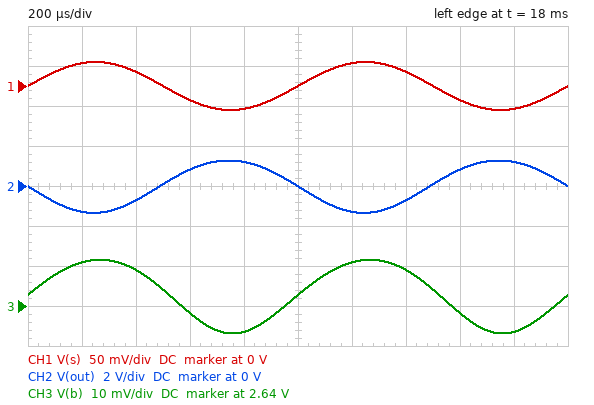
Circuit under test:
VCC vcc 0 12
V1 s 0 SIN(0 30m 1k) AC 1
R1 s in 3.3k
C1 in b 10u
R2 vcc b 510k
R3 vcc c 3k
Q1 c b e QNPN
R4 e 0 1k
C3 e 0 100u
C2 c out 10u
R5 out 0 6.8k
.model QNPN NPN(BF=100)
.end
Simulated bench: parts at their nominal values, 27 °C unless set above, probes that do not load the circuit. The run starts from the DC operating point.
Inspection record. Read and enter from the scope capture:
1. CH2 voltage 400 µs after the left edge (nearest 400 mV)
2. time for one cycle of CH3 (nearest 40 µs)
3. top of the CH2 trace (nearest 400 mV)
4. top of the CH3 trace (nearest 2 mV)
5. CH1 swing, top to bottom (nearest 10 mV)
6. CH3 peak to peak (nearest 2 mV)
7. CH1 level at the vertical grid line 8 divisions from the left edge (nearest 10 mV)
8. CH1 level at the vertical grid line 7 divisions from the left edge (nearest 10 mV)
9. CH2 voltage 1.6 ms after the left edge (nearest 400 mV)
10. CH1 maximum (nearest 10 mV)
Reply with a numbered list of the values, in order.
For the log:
1. -800 mV
2. 1.00 ms
3. 1.2 V
4. 2.652 V
5. 60 mV
6. 18 mV
7. -20 mV
8. 20 mV
9. 800 mV
10. 30 mV
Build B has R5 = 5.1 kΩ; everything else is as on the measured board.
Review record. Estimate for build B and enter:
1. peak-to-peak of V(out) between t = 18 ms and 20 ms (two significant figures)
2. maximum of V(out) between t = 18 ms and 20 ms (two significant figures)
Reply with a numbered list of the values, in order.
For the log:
1. 2.4 V
2. 1.2 V
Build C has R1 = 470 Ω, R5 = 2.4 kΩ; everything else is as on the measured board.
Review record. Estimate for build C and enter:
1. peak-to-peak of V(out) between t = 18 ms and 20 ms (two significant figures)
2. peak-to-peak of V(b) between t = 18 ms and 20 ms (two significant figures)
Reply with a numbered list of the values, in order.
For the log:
1. 3.9 V
2. 46 mV
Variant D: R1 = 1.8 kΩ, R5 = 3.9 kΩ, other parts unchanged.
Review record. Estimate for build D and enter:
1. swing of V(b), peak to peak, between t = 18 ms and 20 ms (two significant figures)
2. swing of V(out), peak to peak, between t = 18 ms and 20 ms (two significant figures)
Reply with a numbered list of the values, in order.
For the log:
1. 27 mV
2. 3.1 V
